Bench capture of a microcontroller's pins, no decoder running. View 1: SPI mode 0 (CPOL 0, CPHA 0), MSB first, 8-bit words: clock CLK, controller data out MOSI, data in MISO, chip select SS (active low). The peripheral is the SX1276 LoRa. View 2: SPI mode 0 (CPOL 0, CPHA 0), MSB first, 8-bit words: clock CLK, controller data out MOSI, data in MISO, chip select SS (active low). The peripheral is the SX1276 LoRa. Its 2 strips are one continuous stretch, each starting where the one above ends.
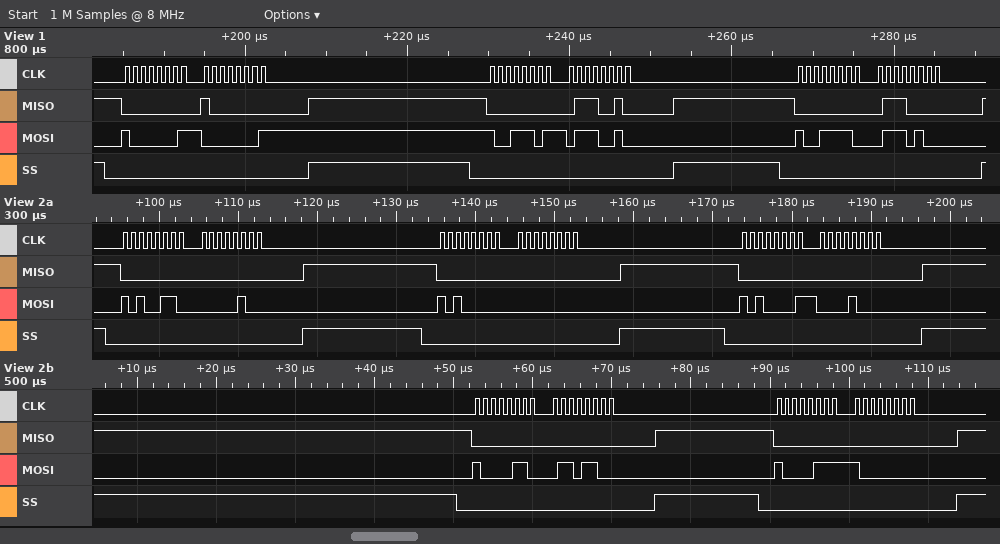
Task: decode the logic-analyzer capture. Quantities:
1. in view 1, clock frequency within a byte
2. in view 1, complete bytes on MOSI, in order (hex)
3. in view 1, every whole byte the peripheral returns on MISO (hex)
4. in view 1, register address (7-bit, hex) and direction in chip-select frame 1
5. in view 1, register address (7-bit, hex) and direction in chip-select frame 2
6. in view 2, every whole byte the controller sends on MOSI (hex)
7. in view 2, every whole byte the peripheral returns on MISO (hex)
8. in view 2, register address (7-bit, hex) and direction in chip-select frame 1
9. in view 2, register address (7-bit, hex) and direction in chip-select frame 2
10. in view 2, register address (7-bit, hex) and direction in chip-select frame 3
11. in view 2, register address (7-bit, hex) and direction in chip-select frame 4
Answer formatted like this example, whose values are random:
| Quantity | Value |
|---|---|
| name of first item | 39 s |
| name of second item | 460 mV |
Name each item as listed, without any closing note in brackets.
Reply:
| Quantity | Value |
|---|---|
| in view 1, clock frequency within a byte | 1 MHz |
| in view 1, complete bytes on MOSI, in order | 0x81 0x01 0x9D 0x72 0x9E 0x74 |
| in view 1, every whole byte the peripheral returns on MISO | 0x00 0x80 0x00 0x72 0x00 0x70 |
| in view 1, register address (7-bit, hex) and direction in chip-select frame 1 | 0x01 write |
| in view 1, register address (7-bit, hex) and direction in chip-select frame 2 | 0x1D write |
| in view 2, every whole byte the controller sends on MOSI | A6 04 A0 00 A1 08 86 6C 87 80 |
| in view 2, every whole byte the peripheral returns on MISO | 00 00 00 00 00 00 00 00 00 00 |
| in view 2, register address (7-bit, hex) and direction in chip-select frame 1 | 0x26 write |
| in view 2, register address (7-bit, hex) and direction in chip-select frame 2 | 0x20 write |
| in view 2, register address (7-bit, hex) and direction in chip-select frame 3 | 0x21 write |
| in view 2, register address (7-bit, hex) and direction in chip-select frame 4 | 0x06 write |
